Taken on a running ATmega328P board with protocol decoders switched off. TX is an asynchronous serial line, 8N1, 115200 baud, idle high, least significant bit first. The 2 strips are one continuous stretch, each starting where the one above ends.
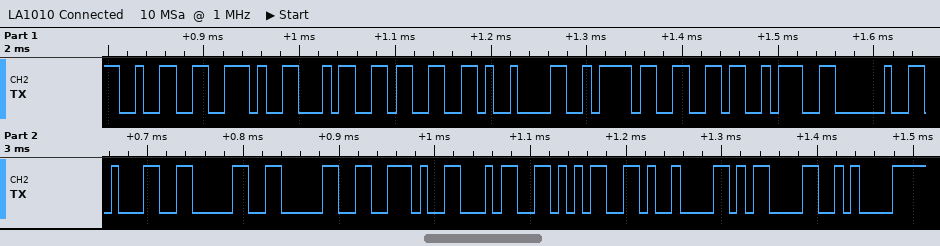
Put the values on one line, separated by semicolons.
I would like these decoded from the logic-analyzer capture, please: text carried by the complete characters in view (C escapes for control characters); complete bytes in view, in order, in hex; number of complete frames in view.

"2.43\tzf: 100.45\t\r\n"; 32 2E 34 33 09 7A 66 3A 20 31 30 30 2E 34 35 09 0D 0A; 18
